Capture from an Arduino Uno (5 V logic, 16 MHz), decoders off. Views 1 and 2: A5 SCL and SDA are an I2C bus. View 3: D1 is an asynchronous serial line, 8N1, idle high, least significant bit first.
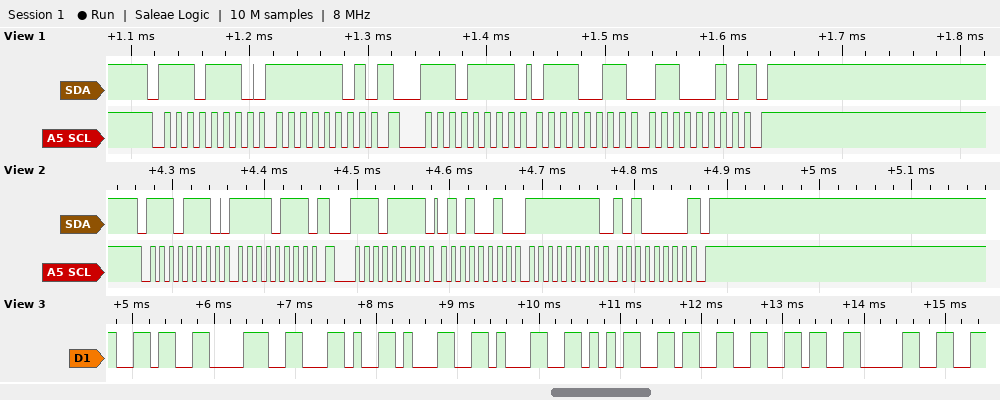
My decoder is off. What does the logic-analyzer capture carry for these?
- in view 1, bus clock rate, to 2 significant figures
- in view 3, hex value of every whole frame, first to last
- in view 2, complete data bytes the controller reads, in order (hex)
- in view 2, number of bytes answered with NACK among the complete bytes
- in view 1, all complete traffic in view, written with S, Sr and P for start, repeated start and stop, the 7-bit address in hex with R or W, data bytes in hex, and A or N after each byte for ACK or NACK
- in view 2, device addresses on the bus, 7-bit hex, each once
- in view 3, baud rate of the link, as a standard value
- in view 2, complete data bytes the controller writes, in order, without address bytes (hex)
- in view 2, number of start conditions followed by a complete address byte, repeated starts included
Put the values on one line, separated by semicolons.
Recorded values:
100 kHz; 36 38 2C 31 31 35 33 36 30; 52 FF A0; 1; S 77W A FD A Sr 77R A 73 A 62 N P; 0x77; 9600 baud; F7; 2
